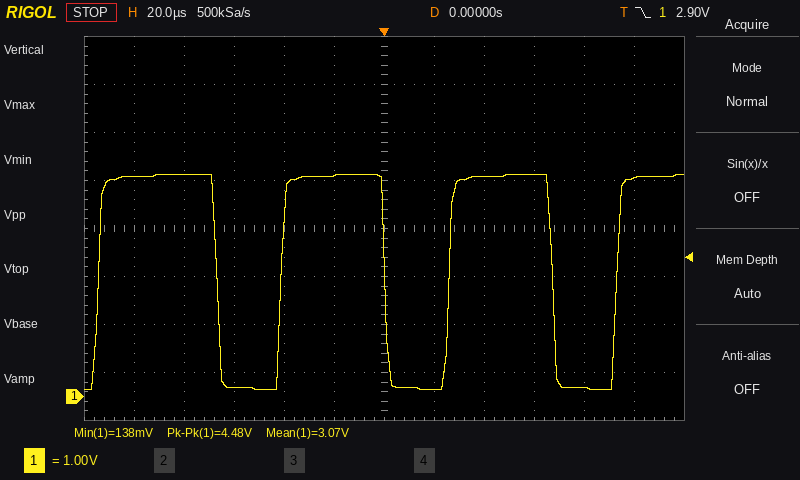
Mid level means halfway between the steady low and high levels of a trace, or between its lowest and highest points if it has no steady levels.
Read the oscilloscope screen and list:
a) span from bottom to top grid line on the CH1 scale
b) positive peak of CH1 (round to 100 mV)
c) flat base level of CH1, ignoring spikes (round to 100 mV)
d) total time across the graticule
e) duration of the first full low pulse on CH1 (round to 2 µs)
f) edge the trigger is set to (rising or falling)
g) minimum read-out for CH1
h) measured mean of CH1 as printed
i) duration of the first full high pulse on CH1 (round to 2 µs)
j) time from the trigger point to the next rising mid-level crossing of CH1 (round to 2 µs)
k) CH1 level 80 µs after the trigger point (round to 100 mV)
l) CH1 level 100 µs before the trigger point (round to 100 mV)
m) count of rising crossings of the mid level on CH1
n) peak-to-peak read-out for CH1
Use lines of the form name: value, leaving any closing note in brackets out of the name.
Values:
span from bottom to top grid line on the CH1 scale: 8 V
positive peak of CH1: 4.6 V
flat base level of CH1, ignoring spikes: 200 mV
total time across the graticule: 240 µs
duration of the first full low pulse on CH1: 26 µs
edge the trigger is set to: falling
minimum read-out for CH1: 138 mV
measured mean of CH1 as printed: 3.07 V
duration of the first full high pulse on CH1: 48 µs
time from the trigger point to the next rising mid-level crossing of CH1: 26 µs
CH1 level 80 µs after the trigger point: 200 mV
CH1 level 100 µs before the trigger point: 4.6 V
count of rising crossings of the mid level on CH1: 4
peak-to-peak read-out for CH1: 4.48 V
